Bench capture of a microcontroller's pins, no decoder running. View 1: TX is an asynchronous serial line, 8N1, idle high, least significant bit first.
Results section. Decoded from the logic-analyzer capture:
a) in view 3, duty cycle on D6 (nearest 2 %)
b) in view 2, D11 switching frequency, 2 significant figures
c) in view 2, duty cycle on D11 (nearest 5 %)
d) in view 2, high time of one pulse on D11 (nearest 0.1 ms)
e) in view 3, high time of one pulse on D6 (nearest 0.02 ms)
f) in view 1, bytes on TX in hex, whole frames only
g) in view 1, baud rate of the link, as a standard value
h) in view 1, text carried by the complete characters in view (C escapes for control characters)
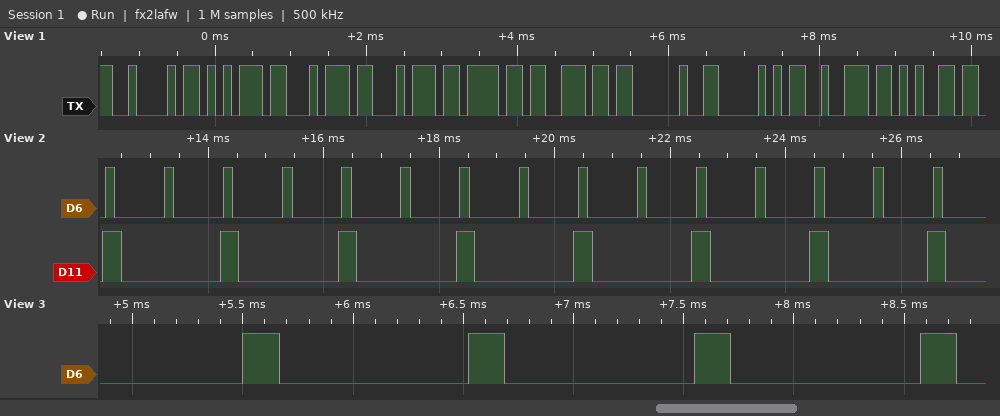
16 %
490 Hz
15 %
0.3 ms
0.16 ms
42 75 74 74 6F 6E 20 50 72 65
9600 baud
"Button Pre"
